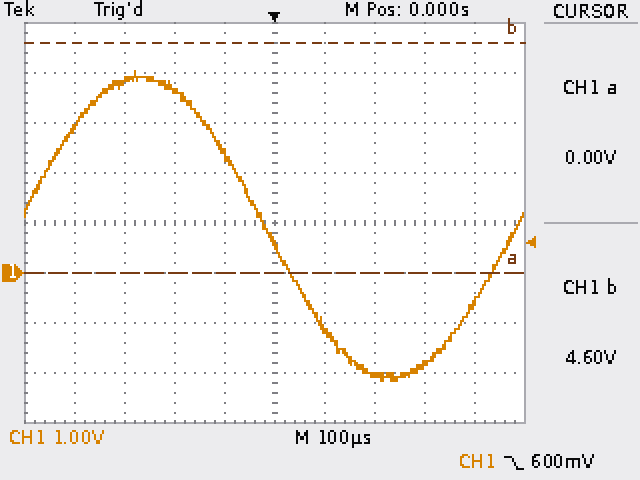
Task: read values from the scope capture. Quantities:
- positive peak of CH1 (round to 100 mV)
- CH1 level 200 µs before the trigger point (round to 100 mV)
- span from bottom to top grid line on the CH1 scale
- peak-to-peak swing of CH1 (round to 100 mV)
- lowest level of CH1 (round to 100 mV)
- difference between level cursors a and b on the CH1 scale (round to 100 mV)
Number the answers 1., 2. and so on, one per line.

1. 4.0 V
2. 3.7 V
3. 8 V
4. 6.2 V
5. -2.2 V
6. 4.6 V
